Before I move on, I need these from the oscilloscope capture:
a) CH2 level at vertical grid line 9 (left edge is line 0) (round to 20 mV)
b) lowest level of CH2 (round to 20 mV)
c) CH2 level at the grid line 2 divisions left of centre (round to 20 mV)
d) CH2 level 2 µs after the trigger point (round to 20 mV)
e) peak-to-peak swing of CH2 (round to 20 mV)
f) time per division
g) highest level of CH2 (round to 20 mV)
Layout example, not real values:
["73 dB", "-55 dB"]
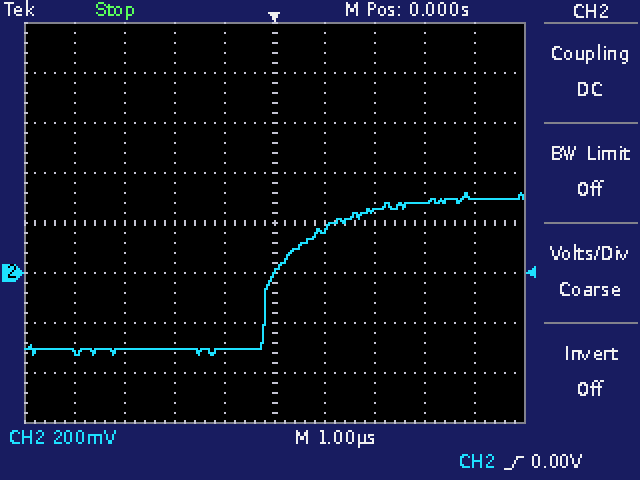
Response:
["300 mV", "-320 mV", "-300 mV", "240 mV", "640 mV", "1 µs", "320 mV"]
